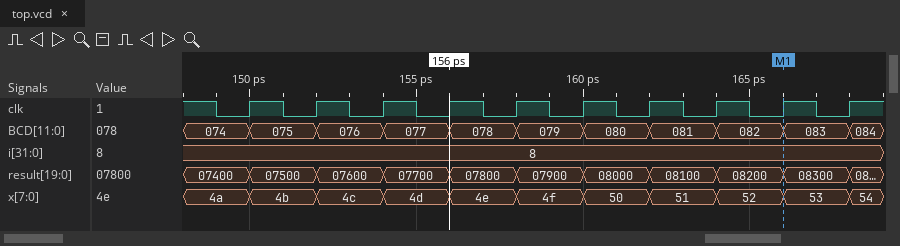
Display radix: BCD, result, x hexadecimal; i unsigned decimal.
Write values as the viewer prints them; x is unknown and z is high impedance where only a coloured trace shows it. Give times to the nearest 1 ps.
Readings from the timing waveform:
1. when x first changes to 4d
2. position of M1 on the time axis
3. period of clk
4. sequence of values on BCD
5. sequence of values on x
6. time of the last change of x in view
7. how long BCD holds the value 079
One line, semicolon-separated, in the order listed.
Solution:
154 ps; 166 ps; 2 ps; 074, 075, 076, 077, 078, 079, 080, 081, 082, 083, 084; 4a, 4b, 4c, 4d, 4e, 4f, 50, 51, 52, 53, 54; 168 ps; 2 ps
